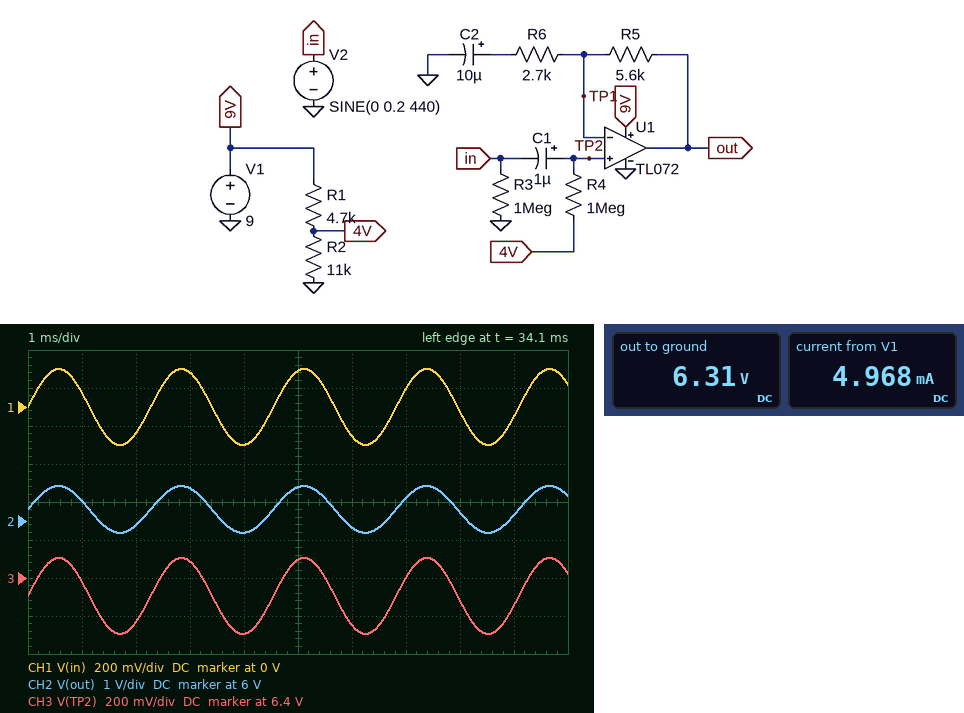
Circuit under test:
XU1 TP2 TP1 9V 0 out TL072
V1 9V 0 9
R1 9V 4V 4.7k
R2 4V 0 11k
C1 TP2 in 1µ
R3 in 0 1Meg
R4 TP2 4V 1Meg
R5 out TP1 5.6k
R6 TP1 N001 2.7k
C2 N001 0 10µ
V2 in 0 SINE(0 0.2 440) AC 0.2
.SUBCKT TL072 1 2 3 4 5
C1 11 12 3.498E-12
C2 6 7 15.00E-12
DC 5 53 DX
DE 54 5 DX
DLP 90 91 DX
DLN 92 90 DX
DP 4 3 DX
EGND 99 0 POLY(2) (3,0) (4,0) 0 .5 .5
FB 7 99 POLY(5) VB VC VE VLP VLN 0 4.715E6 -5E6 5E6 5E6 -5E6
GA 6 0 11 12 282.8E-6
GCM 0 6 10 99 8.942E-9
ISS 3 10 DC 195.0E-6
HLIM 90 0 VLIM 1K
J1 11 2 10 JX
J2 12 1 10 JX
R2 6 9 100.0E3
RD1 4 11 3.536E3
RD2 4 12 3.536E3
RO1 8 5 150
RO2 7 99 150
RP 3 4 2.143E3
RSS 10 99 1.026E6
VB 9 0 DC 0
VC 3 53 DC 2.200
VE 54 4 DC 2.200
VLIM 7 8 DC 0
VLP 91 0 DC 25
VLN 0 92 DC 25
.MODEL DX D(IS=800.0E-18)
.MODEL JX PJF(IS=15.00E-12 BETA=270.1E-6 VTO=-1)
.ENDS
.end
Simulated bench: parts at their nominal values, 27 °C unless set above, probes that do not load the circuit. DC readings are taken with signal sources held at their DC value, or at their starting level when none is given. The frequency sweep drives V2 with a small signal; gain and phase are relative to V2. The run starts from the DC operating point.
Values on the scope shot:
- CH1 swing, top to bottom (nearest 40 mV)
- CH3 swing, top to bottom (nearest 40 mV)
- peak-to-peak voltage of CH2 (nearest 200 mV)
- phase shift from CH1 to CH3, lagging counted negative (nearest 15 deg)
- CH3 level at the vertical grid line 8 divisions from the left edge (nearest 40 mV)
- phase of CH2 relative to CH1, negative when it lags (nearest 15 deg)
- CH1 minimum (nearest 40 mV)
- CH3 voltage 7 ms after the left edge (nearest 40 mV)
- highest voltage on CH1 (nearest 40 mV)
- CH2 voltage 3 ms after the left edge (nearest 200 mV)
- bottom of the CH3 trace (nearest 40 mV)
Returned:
400 mV
400 mV
1.2 V
0 deg
6.28 V
0 deg
-200 mV
6.40 V
200 mV
6.8 V
6.12 V
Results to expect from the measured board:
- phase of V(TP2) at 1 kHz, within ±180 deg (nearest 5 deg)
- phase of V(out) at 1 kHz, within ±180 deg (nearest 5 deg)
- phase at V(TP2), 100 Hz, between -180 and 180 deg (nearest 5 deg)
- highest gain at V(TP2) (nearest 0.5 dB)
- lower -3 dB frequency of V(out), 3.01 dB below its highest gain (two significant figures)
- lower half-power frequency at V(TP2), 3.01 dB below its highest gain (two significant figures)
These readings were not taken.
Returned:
0 deg
0 deg
0 deg
0 dB
5.2 Hz
160 mHz
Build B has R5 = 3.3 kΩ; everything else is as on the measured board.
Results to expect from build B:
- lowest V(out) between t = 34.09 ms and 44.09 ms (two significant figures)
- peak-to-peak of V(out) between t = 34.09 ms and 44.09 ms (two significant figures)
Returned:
5.9 V
890 mV
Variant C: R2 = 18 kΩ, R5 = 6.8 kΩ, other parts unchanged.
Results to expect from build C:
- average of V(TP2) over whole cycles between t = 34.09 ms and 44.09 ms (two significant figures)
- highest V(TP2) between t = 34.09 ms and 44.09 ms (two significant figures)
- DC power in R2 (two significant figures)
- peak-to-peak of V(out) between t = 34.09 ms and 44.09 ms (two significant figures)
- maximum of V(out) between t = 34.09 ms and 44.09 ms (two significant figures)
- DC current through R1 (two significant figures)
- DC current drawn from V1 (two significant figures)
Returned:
7.1 V
7.3 V
2.8 mW
950 mV
7.4 V
400 µA
4.8 mA
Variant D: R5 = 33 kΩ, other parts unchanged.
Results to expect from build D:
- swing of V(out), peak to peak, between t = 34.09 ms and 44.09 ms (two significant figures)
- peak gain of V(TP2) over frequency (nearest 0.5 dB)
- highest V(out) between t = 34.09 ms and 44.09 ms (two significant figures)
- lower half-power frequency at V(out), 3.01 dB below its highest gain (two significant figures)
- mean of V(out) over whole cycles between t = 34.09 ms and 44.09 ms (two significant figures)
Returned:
3.5 V
0 dB
7.4 V
5.9 Hz
6.1 V
